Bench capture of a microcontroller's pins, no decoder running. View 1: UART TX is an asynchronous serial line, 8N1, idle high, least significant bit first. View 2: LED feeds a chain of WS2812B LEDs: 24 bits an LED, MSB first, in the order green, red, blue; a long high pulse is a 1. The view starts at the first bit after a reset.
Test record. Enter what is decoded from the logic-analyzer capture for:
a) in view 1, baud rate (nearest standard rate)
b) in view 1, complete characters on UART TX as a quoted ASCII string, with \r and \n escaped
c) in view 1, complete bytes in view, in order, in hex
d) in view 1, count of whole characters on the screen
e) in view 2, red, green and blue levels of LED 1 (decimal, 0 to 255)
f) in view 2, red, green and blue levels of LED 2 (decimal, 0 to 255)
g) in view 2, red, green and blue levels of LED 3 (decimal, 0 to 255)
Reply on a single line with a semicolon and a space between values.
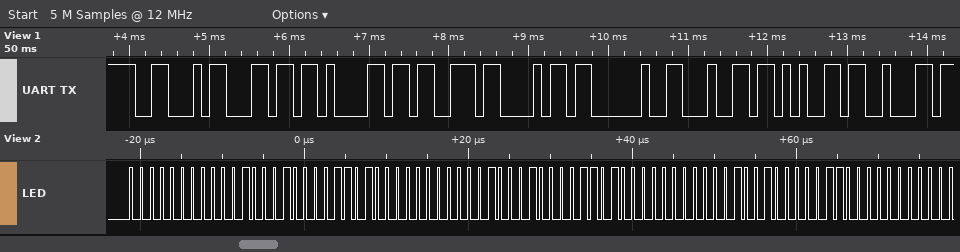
9600 baud; "Flash deb"; 46 6C 61 73 68 20 64 65 62; 9; 17, 0, 13; 17, 0, 13; 18, 0, 12
